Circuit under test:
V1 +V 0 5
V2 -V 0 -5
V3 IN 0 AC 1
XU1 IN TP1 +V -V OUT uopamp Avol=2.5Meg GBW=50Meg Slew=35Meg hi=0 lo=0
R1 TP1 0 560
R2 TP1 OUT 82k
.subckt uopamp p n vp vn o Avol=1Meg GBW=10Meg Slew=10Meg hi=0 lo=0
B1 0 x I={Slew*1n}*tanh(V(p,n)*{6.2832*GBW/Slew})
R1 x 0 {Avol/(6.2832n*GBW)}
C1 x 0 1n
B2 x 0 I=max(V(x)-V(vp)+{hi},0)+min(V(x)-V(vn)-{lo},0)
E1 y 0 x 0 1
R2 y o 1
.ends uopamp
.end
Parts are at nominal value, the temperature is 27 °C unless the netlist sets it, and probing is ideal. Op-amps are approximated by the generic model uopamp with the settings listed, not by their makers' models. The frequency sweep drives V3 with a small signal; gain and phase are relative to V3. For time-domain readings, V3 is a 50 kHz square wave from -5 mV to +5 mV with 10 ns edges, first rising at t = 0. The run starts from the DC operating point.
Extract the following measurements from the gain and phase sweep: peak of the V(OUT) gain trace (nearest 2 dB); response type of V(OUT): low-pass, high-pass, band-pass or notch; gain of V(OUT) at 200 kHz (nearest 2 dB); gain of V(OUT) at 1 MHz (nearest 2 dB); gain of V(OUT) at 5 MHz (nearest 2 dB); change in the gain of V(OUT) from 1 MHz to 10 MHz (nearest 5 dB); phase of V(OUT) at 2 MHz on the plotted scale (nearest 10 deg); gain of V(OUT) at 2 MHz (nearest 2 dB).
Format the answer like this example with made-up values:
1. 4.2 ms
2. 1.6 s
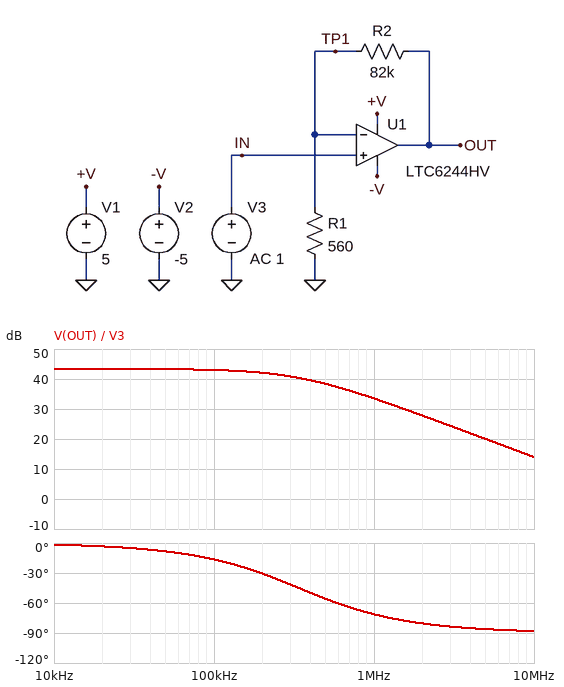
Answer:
1. 44 dB
2. low-pass
3. 42 dB
4. 34 dB
5. 20 dB
6. -20 dB
7. -80 deg
8. 28 dB
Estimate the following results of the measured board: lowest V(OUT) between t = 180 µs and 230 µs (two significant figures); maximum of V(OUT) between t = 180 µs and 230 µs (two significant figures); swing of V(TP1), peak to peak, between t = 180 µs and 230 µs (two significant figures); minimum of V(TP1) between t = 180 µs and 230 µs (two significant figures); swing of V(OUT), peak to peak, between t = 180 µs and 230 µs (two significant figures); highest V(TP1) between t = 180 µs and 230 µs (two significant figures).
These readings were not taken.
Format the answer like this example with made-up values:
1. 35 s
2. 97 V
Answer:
1. -740 mV
2. 740 mV
3. 10 mV
4. -5.0 mV
5. 1.5 V
6. 5.0 mV
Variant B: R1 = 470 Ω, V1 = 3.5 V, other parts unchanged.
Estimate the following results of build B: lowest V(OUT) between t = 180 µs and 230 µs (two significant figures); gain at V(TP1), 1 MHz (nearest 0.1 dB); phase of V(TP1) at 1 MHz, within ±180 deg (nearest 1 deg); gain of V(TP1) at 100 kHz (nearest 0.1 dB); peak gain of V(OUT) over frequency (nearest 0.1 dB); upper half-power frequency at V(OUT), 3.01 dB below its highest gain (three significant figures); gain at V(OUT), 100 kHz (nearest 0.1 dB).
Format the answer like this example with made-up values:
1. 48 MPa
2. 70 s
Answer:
1. -880 mV
2. -11.2 dB
3. -74 deg
4. -0.5 dB
5. 44.9 dB
6. 285 kHz
7. 44.4 dB
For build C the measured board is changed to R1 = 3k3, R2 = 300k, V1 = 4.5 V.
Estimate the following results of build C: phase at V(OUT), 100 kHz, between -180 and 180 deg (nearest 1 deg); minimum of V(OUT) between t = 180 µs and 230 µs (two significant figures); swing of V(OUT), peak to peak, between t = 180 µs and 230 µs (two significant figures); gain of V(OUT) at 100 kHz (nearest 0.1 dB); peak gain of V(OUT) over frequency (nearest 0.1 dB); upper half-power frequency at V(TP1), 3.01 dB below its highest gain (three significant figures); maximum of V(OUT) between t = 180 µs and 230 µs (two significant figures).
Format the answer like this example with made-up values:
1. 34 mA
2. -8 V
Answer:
1. -10 deg
2. -460 mV
3. 920 mV
4. 39.1 dB
5. 39.3 dB
6. 544 kHz
7. 460 mV
